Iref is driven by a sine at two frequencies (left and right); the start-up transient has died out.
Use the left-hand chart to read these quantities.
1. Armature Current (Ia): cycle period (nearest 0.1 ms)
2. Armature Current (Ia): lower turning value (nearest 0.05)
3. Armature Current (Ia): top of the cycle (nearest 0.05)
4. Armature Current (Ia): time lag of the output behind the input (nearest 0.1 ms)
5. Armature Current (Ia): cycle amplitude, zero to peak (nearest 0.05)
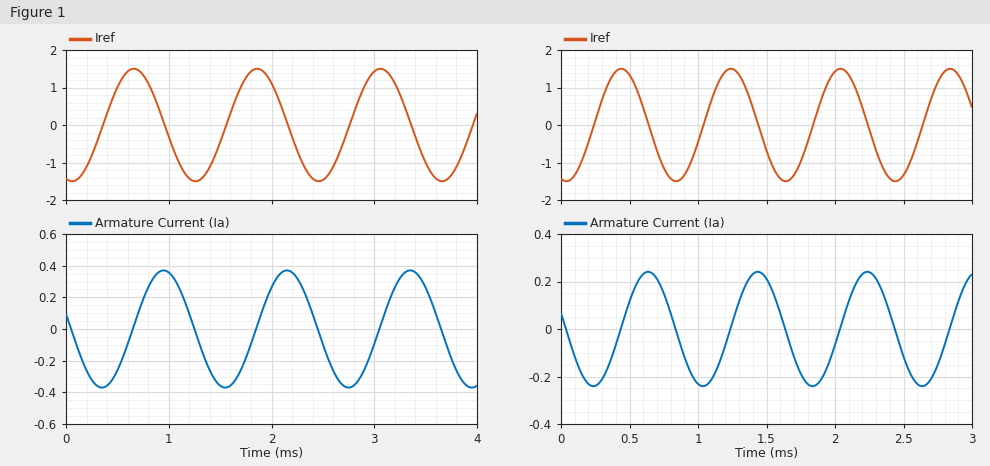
1.2 ms
-0.35
0.35
0.3 ms
0.35
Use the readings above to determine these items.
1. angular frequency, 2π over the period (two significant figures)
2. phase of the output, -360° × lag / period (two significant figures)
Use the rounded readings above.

5.2 rad/ms
-90°
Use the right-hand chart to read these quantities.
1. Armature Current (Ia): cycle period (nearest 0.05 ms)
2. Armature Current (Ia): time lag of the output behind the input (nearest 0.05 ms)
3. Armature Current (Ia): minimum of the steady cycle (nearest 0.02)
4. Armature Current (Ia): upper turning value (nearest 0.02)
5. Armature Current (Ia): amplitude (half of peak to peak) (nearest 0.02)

0.80 ms
0.20 ms
-0.24
0.24
0.24
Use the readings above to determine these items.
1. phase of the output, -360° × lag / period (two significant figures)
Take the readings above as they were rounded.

-90°
